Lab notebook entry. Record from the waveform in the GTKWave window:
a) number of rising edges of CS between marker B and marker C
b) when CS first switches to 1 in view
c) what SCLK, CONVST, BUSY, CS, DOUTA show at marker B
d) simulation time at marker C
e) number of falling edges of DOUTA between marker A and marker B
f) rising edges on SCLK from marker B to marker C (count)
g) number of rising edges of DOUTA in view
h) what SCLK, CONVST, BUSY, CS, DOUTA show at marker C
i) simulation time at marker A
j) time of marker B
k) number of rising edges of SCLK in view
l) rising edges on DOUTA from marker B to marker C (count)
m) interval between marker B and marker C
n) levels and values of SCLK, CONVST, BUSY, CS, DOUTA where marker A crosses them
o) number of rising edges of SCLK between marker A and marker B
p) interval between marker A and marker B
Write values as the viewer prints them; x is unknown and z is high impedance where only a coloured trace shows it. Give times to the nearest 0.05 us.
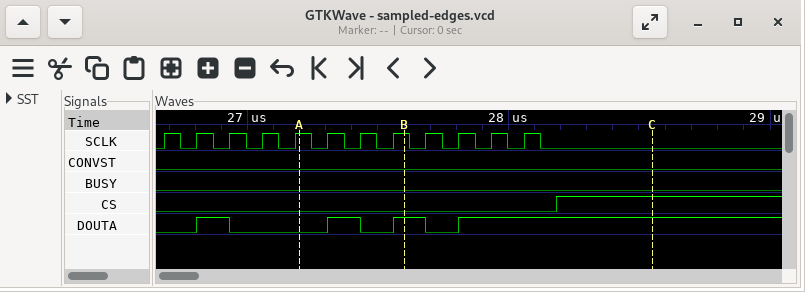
1
28.2 us
SCLK=1, CONVST=0, BUSY=0, CS=0, DOUTA=1
28.55 us
1
4
4
SCLK=0, CONVST=0, BUSY=0, CS=1, DOUTA=1
27.2 us
27.6 us
12
1
0.95 us
SCLK=1, CONVST=0, BUSY=0, CS=0, DOUTA=0
3
0.4 us
